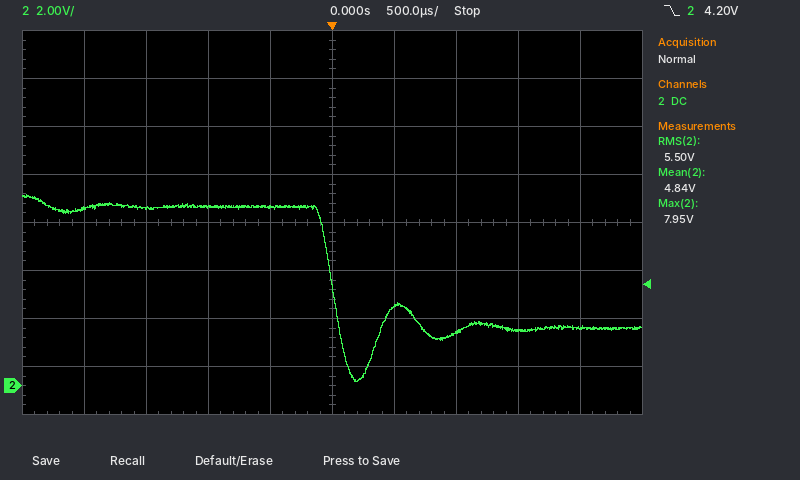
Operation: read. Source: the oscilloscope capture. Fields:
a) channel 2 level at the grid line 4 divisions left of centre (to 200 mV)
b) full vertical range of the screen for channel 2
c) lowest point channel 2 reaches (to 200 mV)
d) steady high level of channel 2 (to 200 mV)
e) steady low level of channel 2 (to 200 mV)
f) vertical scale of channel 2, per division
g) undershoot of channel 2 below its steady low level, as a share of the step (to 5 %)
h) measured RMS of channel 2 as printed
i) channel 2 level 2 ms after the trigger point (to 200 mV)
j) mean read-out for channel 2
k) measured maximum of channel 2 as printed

7.4 V
16 V
200 mV
7.4 V
2.4 V
2 V
45 %
5.50 V
2.4 V
4.84 V
7.95 V
